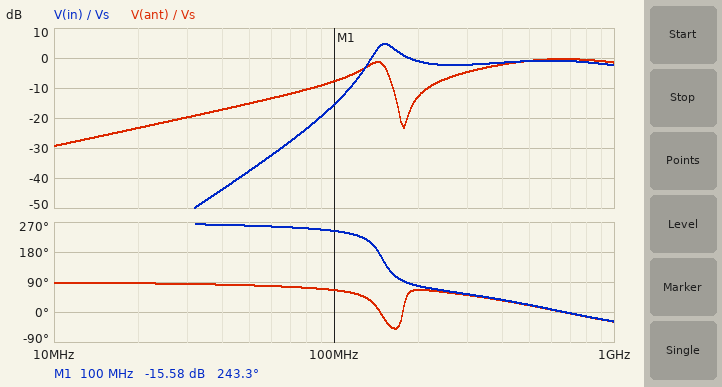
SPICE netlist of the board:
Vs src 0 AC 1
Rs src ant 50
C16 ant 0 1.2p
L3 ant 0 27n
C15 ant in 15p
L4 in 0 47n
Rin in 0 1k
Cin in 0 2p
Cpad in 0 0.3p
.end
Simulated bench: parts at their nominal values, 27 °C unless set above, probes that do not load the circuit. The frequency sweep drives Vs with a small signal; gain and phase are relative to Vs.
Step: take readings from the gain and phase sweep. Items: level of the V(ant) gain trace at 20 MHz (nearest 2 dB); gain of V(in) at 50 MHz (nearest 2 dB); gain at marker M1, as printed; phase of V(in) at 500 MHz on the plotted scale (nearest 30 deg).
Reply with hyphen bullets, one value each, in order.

- -24 dB
- -38 dB
- -15.58 dB
- 30 deg
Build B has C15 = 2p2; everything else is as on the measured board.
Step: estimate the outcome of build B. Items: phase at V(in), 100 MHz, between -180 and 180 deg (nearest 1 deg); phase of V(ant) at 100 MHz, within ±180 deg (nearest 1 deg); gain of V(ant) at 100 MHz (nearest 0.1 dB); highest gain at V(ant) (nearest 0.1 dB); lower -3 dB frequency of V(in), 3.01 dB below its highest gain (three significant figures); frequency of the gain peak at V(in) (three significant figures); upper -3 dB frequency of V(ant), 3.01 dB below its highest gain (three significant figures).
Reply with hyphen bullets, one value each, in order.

- -111 deg
- 71 deg
- -9.6 dB
- -0.2 dB
- 312 MHz
- 339 MHz
- 1.68 GHz
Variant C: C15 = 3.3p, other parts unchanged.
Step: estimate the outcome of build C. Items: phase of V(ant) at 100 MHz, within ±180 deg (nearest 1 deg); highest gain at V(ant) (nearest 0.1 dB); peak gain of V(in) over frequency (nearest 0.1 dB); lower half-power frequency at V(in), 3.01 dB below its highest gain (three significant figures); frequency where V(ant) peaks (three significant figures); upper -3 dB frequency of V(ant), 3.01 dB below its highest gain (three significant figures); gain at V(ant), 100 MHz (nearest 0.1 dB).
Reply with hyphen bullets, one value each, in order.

- 70 deg
- -0.2 dB
- 6.8 dB
- 272 MHz
- 692 MHz
- 1.57 GHz
- -9.5 dB
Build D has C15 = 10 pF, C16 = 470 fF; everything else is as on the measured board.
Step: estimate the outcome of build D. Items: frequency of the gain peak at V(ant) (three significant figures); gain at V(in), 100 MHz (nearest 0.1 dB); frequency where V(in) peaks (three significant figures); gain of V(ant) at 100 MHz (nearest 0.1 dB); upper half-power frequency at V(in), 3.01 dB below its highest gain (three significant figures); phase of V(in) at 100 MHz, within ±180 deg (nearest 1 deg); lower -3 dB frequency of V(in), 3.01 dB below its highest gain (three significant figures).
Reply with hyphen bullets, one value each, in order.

- 760 MHz
- -21.1 dB
- 185 MHz
- -8.7 dB
- 212 MHz
- -114 deg
- 170 MHz
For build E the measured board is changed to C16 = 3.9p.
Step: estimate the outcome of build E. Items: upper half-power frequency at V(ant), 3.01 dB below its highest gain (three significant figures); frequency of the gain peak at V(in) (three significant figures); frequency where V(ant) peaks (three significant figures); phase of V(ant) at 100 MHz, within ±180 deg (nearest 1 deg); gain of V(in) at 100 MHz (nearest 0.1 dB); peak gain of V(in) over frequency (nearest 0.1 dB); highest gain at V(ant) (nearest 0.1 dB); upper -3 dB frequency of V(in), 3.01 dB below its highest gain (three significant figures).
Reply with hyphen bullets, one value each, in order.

- 845 MHz
- 151 MHz
- 492 MHz
- 65 deg
- -15.3 dB
- 4.4 dB
- -0.4 dB
- 173 MHz
